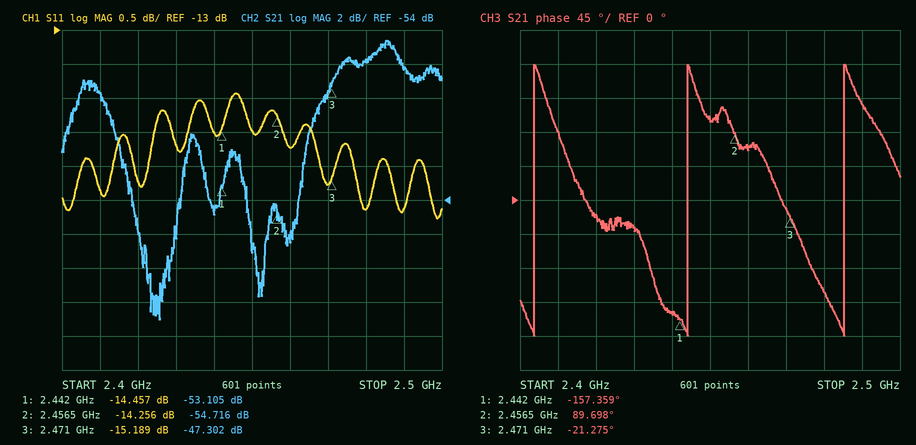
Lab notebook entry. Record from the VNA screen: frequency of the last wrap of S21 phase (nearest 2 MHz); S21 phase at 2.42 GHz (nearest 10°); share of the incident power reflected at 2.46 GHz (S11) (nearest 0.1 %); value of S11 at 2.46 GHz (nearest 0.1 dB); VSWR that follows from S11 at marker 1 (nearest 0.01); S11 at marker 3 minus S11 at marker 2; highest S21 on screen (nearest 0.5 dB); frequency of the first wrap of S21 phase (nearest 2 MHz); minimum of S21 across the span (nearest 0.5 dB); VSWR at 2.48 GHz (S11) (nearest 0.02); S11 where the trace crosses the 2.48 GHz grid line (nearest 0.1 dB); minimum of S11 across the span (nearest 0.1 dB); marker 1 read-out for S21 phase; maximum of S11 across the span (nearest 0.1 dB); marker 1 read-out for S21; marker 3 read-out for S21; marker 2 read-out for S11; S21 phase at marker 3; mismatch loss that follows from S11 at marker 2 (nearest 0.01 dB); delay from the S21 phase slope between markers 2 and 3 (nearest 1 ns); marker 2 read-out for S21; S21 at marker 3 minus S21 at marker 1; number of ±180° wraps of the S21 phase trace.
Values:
2.486 GHz
-20°
3.4 %
-14.7 dB
1.47
-0.933 dB
-44.5 dB
2.404 GHz
-61.0 dB
1.40
-15.6 dB
-15.8 dB
-157.359°
-13.9 dB
-53.105 dB
-47.302 dB
-14.256 dB
-21.275°
0.17 dB
21 ns
-54.716 dB
5.803 dB
3
